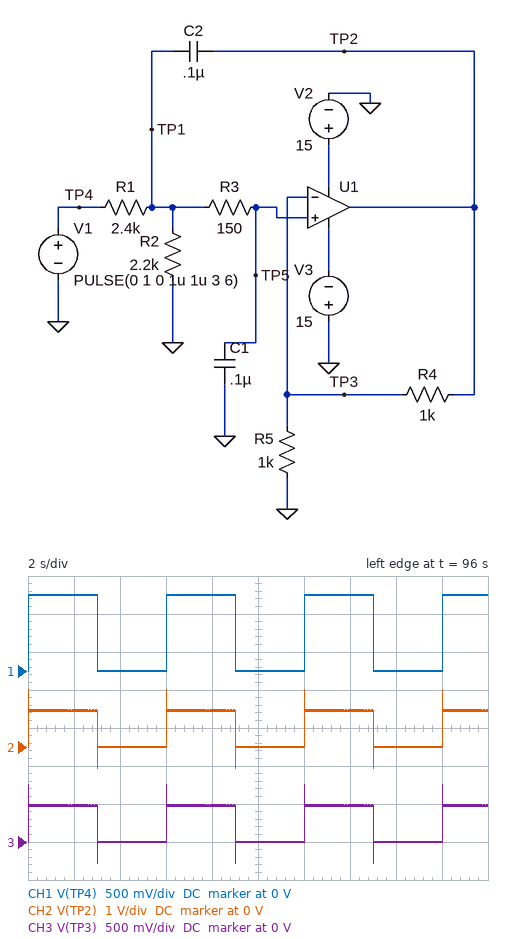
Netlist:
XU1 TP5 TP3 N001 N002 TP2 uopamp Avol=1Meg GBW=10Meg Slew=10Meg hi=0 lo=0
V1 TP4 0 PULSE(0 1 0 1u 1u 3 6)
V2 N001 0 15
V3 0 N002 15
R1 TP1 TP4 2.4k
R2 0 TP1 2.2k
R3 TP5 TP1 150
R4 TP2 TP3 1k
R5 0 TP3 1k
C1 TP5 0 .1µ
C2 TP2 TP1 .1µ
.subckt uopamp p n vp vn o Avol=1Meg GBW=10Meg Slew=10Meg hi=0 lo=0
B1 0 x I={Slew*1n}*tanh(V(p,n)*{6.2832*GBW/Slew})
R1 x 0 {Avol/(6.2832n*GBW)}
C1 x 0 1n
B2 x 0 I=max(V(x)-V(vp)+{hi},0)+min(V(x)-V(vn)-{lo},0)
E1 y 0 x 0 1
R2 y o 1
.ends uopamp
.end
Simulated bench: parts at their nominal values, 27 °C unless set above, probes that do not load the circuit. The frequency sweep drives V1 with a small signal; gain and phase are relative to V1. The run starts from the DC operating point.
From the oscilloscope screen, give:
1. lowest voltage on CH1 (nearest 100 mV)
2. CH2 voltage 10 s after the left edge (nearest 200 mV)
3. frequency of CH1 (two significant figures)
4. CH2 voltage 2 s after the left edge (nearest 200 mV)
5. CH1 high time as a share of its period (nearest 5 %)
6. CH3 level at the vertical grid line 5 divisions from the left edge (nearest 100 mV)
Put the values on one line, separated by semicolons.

0 V; 0 V; 170 mHz; 1.0 V; 50 %; 0 V
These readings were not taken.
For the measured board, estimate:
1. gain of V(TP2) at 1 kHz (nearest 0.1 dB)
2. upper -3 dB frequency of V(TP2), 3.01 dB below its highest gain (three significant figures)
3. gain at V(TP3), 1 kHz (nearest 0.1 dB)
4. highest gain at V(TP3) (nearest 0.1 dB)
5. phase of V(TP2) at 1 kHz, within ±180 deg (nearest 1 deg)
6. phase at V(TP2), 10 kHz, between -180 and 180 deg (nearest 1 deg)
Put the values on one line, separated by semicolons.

0.2 dB; 4.35 kHz; -5.8 dB; 2.6 dB; -6 deg; -171 deg
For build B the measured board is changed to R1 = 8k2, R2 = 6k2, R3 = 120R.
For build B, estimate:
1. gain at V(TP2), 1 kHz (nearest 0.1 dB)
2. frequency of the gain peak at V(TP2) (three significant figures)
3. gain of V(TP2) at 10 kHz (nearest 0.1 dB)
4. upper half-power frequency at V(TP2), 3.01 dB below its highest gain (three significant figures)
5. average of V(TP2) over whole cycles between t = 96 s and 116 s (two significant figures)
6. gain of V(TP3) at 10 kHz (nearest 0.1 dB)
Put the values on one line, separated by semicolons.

0.3 dB; 2.42 kHz; -25.3 dB; 2.63 kHz; 430 mV; -31.3 dB
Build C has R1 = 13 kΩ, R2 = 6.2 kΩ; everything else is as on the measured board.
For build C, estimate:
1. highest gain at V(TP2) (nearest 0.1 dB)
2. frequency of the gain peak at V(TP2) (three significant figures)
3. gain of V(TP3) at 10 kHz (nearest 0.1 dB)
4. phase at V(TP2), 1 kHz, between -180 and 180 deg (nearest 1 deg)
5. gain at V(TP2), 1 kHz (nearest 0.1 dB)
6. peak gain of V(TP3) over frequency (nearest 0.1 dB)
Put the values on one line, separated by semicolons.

10.7 dB; 1.98 kHz; -37.4 dB; -7 deg; -1.4 dB; 4.7 dB
